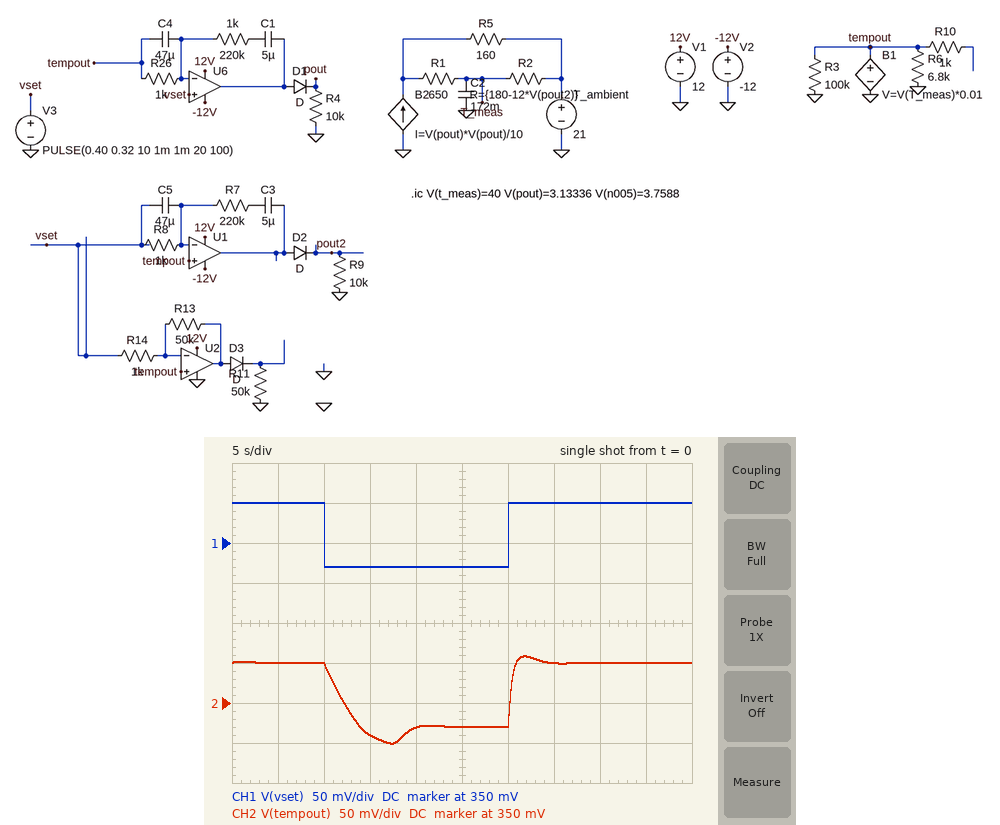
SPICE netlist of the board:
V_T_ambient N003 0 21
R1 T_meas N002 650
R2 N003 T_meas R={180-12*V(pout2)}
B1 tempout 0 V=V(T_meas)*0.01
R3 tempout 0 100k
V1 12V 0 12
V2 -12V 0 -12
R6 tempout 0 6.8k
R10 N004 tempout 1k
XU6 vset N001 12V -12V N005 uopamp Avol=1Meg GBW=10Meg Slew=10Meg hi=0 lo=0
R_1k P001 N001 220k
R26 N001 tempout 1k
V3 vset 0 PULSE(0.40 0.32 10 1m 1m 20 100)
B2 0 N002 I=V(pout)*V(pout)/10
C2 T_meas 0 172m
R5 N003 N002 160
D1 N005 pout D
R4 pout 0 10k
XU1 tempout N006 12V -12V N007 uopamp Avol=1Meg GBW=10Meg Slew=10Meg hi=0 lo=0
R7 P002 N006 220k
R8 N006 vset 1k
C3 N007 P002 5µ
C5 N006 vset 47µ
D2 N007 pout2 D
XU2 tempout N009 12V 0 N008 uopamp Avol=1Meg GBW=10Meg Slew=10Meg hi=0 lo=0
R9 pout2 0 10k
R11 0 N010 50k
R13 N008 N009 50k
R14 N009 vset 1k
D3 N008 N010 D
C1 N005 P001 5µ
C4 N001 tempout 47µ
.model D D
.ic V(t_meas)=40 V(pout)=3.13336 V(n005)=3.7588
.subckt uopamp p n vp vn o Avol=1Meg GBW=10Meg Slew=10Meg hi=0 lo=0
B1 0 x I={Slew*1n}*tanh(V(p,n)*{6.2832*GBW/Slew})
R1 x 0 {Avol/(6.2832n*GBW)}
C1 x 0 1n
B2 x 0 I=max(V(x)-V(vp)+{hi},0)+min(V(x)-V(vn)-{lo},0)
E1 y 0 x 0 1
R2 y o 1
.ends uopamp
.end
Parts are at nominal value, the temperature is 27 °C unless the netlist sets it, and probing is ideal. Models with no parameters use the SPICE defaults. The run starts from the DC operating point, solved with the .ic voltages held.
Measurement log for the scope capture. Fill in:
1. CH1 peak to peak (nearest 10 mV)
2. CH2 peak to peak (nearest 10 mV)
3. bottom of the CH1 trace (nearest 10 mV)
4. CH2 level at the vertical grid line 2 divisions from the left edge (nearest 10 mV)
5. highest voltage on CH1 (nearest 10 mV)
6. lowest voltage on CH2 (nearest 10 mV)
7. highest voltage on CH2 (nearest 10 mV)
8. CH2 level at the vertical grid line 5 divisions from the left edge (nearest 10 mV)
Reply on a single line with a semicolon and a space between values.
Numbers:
80 mV; 110 mV; 320 mV; 400 mV; 400 mV; 300 mV; 410 mV; 320 mV
